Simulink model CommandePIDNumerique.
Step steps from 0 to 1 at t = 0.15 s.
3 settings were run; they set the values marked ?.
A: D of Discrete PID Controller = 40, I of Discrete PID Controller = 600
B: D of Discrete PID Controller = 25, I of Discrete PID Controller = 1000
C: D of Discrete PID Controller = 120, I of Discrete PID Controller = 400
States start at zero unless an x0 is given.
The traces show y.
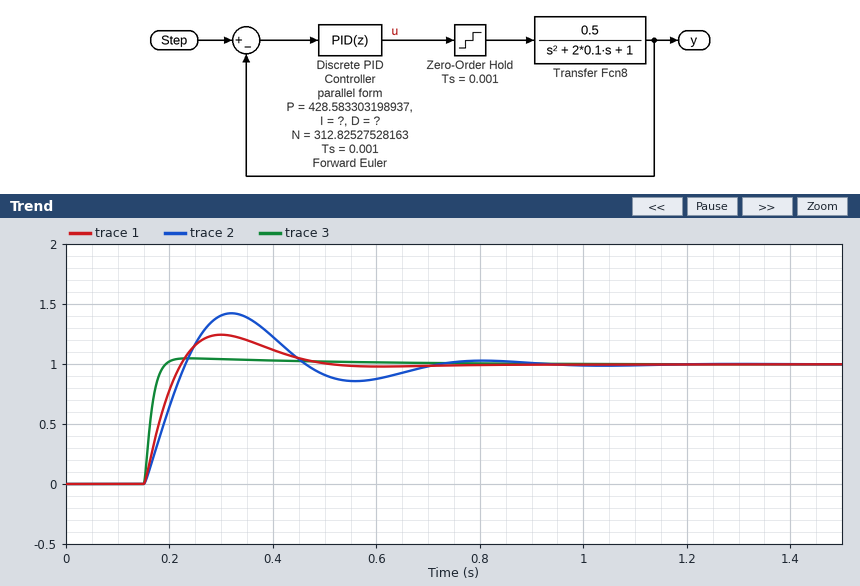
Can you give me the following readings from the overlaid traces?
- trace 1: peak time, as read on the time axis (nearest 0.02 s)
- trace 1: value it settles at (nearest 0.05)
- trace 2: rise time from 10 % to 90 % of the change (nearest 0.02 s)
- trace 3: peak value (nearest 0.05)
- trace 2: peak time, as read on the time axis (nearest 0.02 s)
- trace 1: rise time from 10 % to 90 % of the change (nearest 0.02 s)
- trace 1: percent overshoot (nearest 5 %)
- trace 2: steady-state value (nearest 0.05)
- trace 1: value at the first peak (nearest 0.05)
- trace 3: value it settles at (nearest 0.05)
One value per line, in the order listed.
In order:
0.30 s
1.00
0.06 s
1.05
0.32 s
0.06 s
25 %
1.00
1.25
1.00
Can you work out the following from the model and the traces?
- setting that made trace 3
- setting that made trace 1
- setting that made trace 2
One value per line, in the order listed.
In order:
C
A
B
